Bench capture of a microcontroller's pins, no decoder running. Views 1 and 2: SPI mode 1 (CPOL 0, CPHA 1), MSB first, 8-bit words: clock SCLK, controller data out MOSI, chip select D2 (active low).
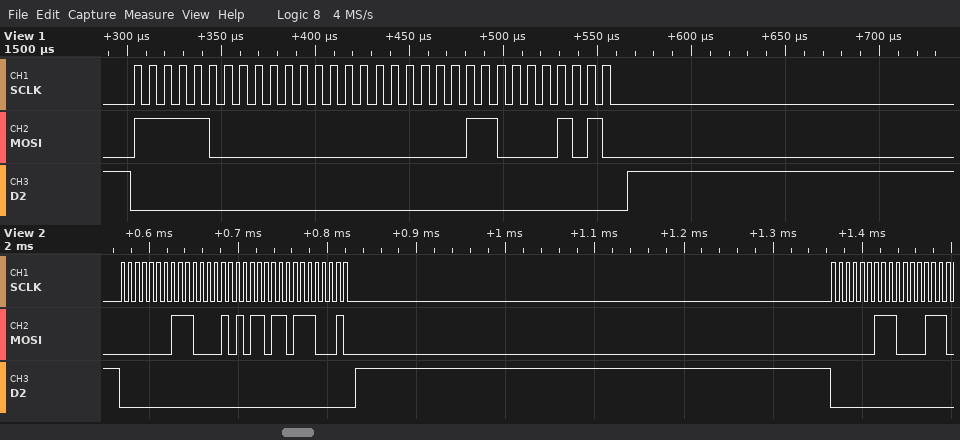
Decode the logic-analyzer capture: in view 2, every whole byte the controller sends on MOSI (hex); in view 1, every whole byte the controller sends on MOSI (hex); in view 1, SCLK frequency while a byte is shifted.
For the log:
0x01 0xC2 0xB6 0xE2 0x03 0x87
F8 00 03 0A
125 kHz
